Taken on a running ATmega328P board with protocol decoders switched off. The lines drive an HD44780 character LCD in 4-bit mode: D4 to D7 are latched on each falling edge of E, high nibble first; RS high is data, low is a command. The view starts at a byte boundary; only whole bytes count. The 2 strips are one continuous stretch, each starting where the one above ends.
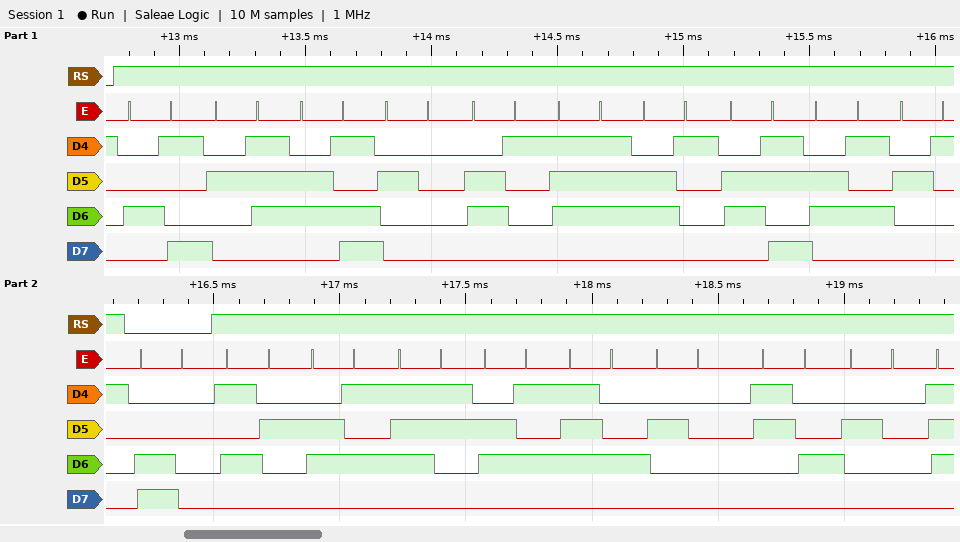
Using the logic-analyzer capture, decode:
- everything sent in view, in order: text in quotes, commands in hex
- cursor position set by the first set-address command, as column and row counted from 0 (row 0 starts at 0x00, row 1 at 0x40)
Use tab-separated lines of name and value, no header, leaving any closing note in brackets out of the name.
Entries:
everything sent in view, in order: text in quotes, commands in hex	"I'm awake!" 0xC0 "Reset 4 "
cursor position set by the first set-address command, as column and row counted from 0	column 0, row 1
